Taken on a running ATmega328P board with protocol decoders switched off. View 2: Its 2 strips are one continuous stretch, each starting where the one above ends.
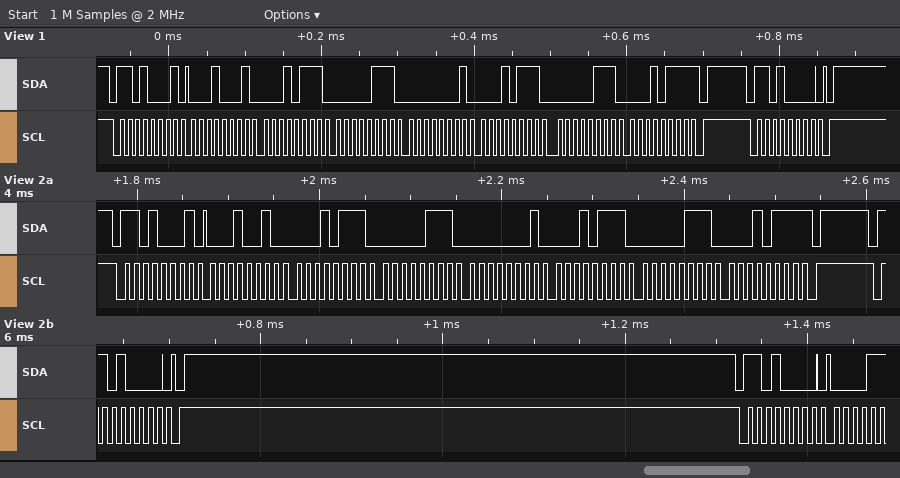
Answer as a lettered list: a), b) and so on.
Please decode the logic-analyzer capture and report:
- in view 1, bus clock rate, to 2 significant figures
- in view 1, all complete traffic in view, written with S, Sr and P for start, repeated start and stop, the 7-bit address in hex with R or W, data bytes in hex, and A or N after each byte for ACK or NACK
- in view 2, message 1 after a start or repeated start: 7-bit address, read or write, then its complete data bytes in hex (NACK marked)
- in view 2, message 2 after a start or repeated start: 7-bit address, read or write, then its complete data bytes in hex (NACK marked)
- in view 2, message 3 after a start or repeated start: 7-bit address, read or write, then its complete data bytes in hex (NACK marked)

a) 100 kHz
b) S 68R A 11 A 17 A 07 A 01 A 17 A 07 A 17 N P S 68W A P
c) 0x68 read: 12 17 07 01 17 07 17 NACK
d) 0x68 write
e) 0x68 write
